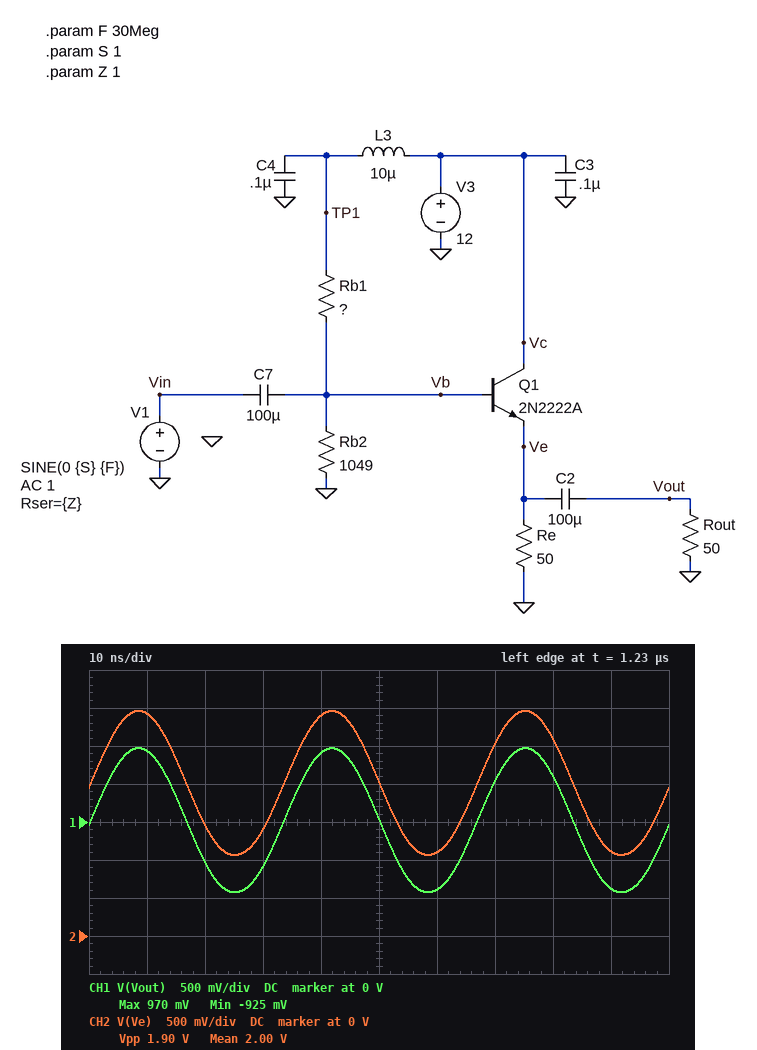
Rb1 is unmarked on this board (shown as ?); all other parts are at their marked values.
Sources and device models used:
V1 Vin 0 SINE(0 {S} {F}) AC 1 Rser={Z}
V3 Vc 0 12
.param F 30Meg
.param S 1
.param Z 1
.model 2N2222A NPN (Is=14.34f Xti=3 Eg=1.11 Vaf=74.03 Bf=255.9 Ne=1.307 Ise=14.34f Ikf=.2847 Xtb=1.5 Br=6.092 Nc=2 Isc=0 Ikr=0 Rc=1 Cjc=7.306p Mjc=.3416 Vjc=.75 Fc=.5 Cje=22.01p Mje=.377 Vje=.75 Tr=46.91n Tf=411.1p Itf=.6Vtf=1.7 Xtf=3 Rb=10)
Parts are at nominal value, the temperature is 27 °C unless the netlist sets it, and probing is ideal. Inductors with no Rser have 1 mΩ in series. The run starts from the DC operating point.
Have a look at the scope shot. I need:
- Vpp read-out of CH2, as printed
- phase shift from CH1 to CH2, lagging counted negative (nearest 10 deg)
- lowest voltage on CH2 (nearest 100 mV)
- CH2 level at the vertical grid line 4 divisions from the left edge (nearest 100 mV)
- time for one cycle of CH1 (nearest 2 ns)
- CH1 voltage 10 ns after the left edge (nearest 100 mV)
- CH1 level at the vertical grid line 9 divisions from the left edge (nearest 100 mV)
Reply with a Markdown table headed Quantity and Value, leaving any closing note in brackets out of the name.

| Quantity | Value |
|---|---|
| Vpp read-out of CH2, as printed | 1.90 V |
| phase shift from CH1 to CH2, lagging counted negative | 0 deg |
| lowest voltage on CH2 | 1.1 V |
| CH2 level at the vertical grid line 4 divisions from the left edge | 2.9 V |
| time for one cycle of CH1 | 34 ns |
| CH1 voltage 10 ns after the left edge | 900 mV |
| CH1 level at the vertical grid line 9 divisions from the left edge | -900 mV |
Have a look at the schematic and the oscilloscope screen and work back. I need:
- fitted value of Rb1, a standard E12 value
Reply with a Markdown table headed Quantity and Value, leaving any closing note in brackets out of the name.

| Quantity | Value |
|---|---|
| fitted value of Rb1, a standard E12 value | 3.3 kΩ |
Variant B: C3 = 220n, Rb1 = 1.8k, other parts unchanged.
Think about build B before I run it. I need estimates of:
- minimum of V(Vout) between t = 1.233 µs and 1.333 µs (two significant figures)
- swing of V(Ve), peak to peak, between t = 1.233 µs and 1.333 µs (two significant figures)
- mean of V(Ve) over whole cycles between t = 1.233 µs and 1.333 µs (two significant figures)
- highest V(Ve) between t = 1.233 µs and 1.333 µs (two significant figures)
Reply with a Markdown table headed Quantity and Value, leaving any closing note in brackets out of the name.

| Quantity | Value |
|---|---|
| minimum of V(Vout) between t = 1.233 µs and 1.333 µs | -970 mV |
| swing of V(Ve), peak to peak, between t = 1.233 µs and 1.333 µs | 1.9 V |
| mean of V(Ve) over whole cycles between t = 1.233 µs and 1.333 µs | 3.4 V |
| highest V(Ve) between t = 1.233 µs and 1.333 µs | 4.4 V |
